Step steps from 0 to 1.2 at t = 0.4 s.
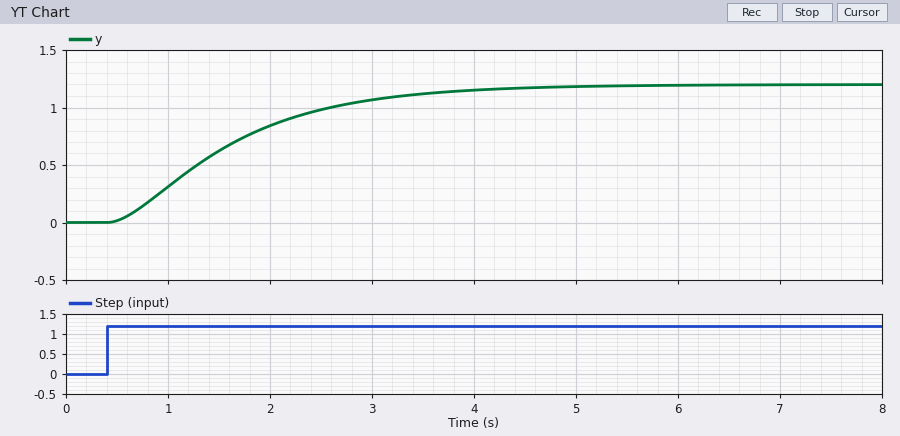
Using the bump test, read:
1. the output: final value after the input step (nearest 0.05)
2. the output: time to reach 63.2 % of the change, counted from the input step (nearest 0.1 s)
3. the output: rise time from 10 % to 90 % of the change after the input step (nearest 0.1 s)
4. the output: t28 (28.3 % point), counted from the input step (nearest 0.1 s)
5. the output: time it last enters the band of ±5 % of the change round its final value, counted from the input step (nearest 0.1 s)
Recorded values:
1.20
1.4 s
2.4 s
0.6 s
3.4 s
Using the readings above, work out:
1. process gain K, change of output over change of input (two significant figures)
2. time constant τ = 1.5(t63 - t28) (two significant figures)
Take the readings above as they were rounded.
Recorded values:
1.0
1.2 s
